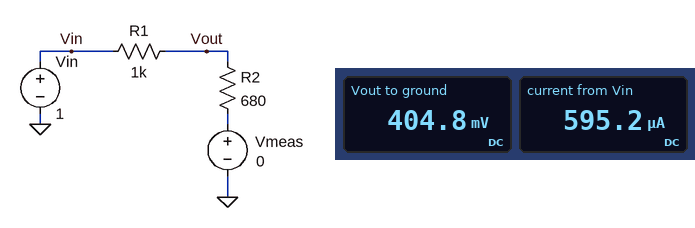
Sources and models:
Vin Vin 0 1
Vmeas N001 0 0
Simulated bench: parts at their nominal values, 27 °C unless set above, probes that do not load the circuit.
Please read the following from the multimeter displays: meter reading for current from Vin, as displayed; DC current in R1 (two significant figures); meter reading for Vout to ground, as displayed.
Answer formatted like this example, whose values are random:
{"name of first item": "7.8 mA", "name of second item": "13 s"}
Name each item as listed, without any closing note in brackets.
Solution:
{"meter reading for current from Vin, as displayed": "595.2 µA", "DC current in R1": "600 µA", "meter reading for Vout to ground, as displayed": "404.8 mV"}
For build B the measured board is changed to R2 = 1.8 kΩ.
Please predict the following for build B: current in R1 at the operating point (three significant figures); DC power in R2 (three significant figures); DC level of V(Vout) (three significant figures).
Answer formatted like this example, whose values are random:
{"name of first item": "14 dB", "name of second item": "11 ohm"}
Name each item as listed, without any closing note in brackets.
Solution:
{"current in R1 at the operating point": "357 µA", "DC power in R2": "230 µW", "DC level of V(Vout)": "643 mV"}
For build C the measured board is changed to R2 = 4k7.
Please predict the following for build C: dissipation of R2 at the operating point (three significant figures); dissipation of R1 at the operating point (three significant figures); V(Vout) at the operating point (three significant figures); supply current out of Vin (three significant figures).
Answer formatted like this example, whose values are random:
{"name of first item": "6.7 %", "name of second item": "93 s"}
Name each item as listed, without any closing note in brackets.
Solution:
{"dissipation of R2 at the operating point": "145 µW", "dissipation of R1 at the operating point": "30.8 µW", "V(Vout) at the operating point": "825 mV", "supply current out of Vin": "175 µA"}
